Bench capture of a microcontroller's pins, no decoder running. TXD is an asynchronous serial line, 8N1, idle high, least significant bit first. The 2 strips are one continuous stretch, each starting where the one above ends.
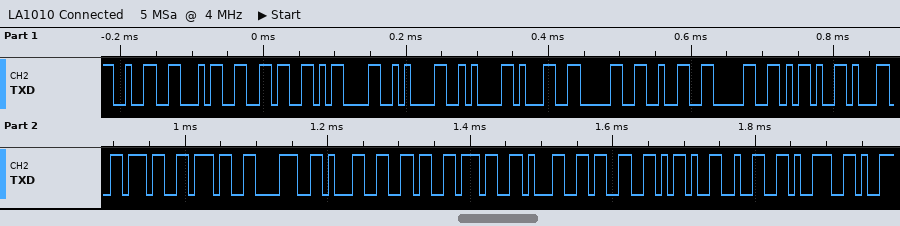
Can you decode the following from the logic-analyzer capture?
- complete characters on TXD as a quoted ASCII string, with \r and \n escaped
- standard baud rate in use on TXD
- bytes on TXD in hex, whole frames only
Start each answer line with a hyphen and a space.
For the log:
- "246\r\n\n1020-177816713-29"
- 115200 baud
- 32 34 36 0D 0A 0A 31 30 32 30 2D 31 37 37 38 31 36 37 31 33 2D 32 39
